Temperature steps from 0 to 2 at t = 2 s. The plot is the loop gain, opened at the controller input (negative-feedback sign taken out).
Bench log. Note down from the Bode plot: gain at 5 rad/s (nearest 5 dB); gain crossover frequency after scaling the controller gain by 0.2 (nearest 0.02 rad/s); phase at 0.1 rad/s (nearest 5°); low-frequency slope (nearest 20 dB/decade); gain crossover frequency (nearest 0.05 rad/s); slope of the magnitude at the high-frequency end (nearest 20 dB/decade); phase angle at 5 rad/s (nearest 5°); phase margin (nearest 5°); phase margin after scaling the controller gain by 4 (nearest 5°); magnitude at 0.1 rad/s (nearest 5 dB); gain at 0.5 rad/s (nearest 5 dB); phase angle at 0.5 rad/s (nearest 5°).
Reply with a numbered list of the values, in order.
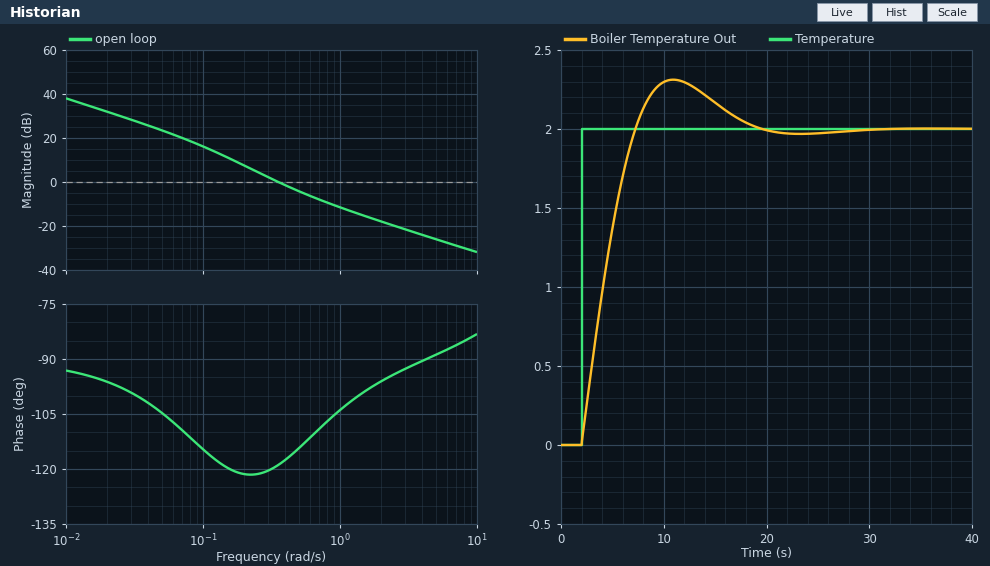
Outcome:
1. -25 dB
2. 0.12 rad/s
3. -115°
4. -20 dB/decade
5. 0.35 rad/s
6. -20 dB/decade
7. -90°
8. 60°
9. 75°
10. 15 dB
11. -5 dB
12. -115°
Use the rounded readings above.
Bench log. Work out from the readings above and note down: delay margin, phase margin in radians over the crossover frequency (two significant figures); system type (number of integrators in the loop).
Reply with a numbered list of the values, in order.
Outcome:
1. 3.0 s
2. 1
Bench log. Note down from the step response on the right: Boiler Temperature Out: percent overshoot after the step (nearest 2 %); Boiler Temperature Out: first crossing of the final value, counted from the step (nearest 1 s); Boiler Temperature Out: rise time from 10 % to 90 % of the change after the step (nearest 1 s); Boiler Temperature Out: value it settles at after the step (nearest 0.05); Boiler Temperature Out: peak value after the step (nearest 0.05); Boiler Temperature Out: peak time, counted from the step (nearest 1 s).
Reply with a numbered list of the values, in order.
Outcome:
1. 16 %
2. 5 s
3. 4 s
4. 2.00
5. 2.30
6. 9 s
